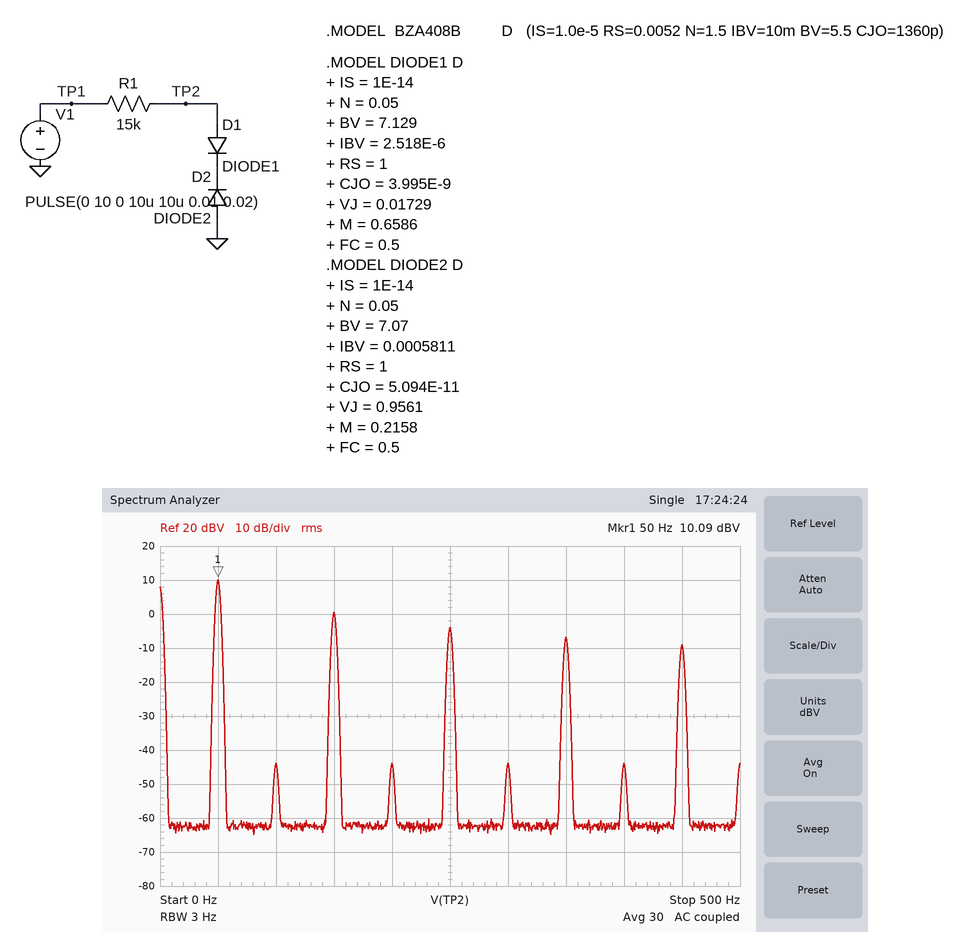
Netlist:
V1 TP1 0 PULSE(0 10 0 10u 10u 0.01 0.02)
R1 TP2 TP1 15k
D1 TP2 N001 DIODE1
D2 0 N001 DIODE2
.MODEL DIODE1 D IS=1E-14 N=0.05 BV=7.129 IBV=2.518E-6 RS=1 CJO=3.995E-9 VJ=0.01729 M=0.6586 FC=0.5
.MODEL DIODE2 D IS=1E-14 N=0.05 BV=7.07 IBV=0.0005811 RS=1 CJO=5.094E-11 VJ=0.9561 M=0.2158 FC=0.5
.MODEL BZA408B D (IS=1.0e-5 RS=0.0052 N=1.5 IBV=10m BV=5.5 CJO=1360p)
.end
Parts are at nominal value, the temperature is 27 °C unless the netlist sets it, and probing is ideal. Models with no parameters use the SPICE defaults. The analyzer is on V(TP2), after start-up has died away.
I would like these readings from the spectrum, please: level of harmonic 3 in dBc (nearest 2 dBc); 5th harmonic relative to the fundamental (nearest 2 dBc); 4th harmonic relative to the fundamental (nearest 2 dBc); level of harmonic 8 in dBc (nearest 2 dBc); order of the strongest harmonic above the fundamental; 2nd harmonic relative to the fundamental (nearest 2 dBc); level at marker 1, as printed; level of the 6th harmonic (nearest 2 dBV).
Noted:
-10 dBc
-14 dBc
-54 dBc
-54 dBc
3
-54 dBc
10.09 dBV
-44 dBV
